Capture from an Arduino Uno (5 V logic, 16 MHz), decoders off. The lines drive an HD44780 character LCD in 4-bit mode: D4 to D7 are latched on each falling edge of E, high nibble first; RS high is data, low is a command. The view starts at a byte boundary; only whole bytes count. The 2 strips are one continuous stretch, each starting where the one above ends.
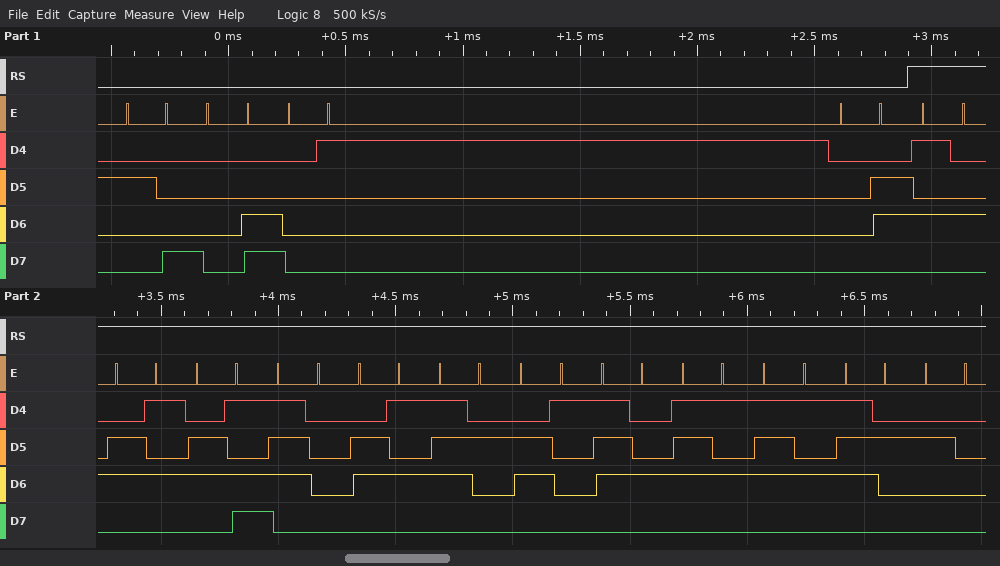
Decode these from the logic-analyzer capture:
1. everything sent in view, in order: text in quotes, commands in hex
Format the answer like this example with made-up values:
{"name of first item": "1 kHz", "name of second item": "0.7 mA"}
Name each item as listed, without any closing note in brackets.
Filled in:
{"everything sent in view, in order: text in quotes, commands in hex": "0x28 0x0C 0x01 0x06 \"Temperatuur \""}
